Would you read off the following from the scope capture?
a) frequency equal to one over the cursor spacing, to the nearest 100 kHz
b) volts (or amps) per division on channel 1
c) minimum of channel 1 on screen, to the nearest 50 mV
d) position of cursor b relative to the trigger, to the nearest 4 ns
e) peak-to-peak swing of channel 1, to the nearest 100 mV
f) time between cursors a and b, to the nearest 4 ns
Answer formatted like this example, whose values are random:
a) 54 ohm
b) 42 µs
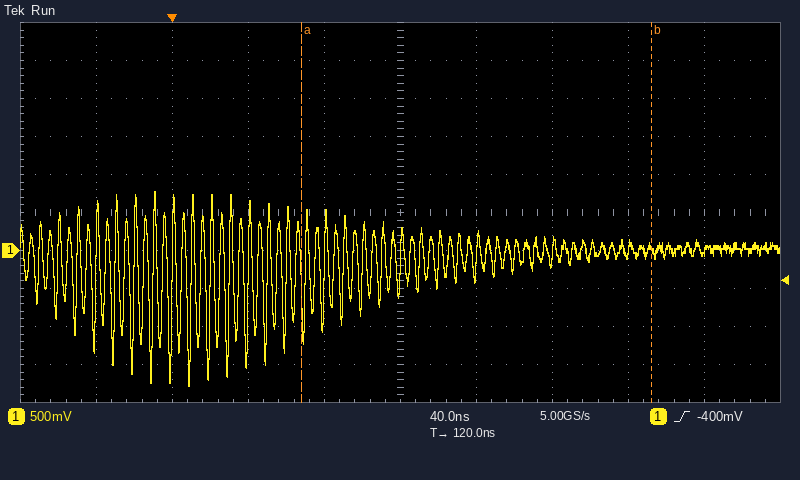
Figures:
a) 5.4 MHz
b) 500 mV
c) -1.80 V
d) +252 ns
e) 2.60 V
f) 184 ns
